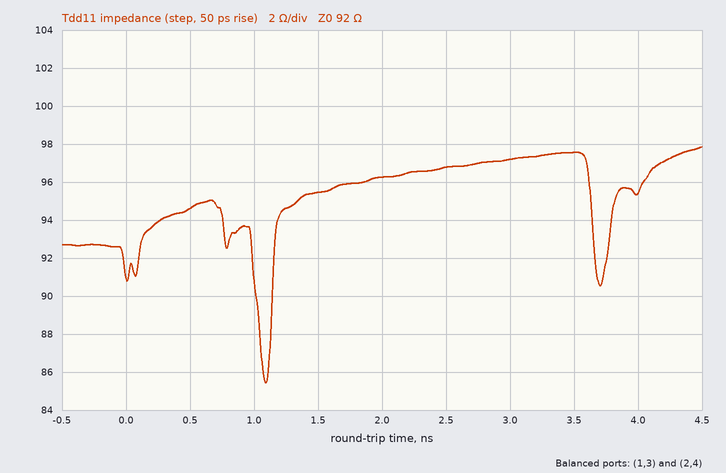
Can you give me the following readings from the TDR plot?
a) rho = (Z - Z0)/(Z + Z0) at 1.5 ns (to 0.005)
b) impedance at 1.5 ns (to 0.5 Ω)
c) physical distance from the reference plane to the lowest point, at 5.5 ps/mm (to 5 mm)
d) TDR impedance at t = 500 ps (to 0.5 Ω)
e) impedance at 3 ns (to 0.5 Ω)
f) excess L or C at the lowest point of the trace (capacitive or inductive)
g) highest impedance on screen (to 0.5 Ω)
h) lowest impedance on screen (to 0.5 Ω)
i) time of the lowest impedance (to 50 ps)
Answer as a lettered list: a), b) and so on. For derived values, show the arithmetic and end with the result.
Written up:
a) (95.5 − 92)/(95.5 + 92) ≈ +0.0187, so +0.020 to the nearest 0.005
b) 95.5 Ω
c) 1.10 ns / 2 / 5.5 ps/mm ≈ 100 mm
d) 94.5 Ω
e) 97.0 Ω
f) capacitive
g) 98.0 Ω
h) 85.5 Ω
i) 1.10 ns
